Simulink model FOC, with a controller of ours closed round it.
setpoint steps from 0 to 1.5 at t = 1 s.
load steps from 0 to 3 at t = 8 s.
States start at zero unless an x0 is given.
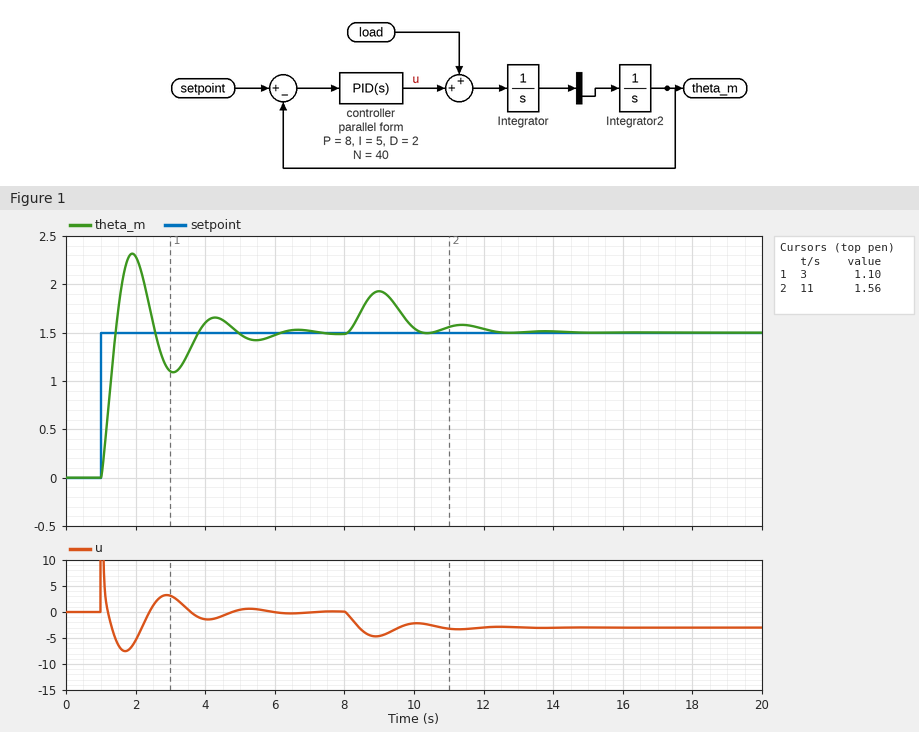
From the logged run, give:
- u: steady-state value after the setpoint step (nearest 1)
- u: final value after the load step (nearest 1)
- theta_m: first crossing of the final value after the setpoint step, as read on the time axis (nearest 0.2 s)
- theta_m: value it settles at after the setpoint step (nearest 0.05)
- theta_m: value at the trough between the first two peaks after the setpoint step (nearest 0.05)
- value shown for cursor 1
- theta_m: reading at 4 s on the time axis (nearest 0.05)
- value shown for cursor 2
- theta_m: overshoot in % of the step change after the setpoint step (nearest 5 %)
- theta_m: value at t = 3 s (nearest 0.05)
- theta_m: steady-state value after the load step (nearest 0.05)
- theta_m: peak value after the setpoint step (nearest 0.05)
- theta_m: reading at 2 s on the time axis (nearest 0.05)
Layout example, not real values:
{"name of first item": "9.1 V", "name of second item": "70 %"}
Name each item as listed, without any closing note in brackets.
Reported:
{"u: steady-state value after the setpoint step": "0", "u: final value after the load step": "-3", "theta_m: first crossing of the final value after the setpoint step, as read on the time axis": "1.4 s", "theta_m: value it settles at after the setpoint step": "1.50", "theta_m: value at the trough between the first two peaks after the setpoint step": "1.10", "value shown for cursor 1": "1.10", "theta_m: reading at 4 s on the time axis": "1.60", "value shown for cursor 2": "1.56", "theta_m: overshoot in % of the step change after the setpoint step": "55 %", "theta_m: value at t = 3 s": "1.10", "theta_m: steady-state value after the load step": "1.50", "theta_m: peak value after the setpoint step": "2.30", "theta_m: reading at 2 s on the time axis": "2.30"}
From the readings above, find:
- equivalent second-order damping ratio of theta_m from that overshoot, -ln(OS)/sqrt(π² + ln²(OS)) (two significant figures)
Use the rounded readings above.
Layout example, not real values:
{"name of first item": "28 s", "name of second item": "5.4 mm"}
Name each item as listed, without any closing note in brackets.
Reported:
{"equivalent second-order damping ratio of theta_m from that overshoot, -ln(OS)/sqrt(π² + ln²(OS))": "0.19"}
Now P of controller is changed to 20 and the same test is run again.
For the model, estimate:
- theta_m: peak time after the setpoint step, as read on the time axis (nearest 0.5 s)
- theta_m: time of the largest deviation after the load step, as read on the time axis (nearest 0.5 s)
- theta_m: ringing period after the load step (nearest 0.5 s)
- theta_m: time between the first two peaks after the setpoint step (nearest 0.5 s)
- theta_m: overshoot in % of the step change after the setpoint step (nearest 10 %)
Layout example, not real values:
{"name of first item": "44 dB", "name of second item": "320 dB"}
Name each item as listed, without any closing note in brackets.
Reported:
{"theta_m: peak time after the setpoint step, as read on the time axis": "1.5 s", "theta_m: time of the largest deviation after the load step, as read on the time axis": "8.5 s", "theta_m: ringing period after the load step": "1.5 s", "theta_m: time between the first two peaks after the setpoint step": "1.5 s", "theta_m: overshoot in % of the step change after the setpoint step": "60 %"}
